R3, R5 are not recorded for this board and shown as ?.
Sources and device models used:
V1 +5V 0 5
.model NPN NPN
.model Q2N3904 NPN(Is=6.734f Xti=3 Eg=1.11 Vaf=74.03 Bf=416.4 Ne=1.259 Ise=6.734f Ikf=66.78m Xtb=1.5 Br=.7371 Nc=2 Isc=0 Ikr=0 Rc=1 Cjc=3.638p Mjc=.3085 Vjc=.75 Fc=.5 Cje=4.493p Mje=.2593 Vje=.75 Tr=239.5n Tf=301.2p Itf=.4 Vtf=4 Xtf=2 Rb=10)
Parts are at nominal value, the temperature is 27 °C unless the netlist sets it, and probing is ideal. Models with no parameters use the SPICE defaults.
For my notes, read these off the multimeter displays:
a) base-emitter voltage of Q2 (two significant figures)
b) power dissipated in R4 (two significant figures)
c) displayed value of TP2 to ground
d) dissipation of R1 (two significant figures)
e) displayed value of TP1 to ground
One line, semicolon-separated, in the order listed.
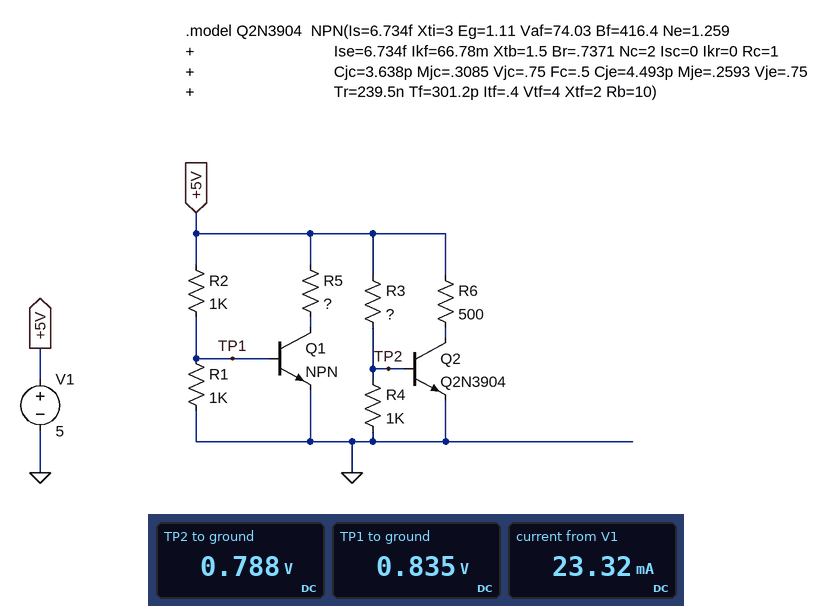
790 mV; 620 µW; 0.788 V; 700 µW; 0.835 V
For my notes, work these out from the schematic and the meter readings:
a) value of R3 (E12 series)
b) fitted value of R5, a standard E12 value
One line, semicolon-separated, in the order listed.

820 Ω; 1.2 kΩ
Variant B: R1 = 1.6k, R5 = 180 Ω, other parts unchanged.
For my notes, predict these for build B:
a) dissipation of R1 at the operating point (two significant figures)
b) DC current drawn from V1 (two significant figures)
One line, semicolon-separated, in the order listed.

470 µW; 47 mA
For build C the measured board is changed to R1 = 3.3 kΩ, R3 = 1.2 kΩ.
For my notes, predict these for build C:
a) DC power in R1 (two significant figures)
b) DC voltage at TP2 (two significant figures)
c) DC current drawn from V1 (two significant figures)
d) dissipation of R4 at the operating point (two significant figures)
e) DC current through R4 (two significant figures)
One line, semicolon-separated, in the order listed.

210 µW; 770 mV; 22 mA; 590 µW; 770 µA
